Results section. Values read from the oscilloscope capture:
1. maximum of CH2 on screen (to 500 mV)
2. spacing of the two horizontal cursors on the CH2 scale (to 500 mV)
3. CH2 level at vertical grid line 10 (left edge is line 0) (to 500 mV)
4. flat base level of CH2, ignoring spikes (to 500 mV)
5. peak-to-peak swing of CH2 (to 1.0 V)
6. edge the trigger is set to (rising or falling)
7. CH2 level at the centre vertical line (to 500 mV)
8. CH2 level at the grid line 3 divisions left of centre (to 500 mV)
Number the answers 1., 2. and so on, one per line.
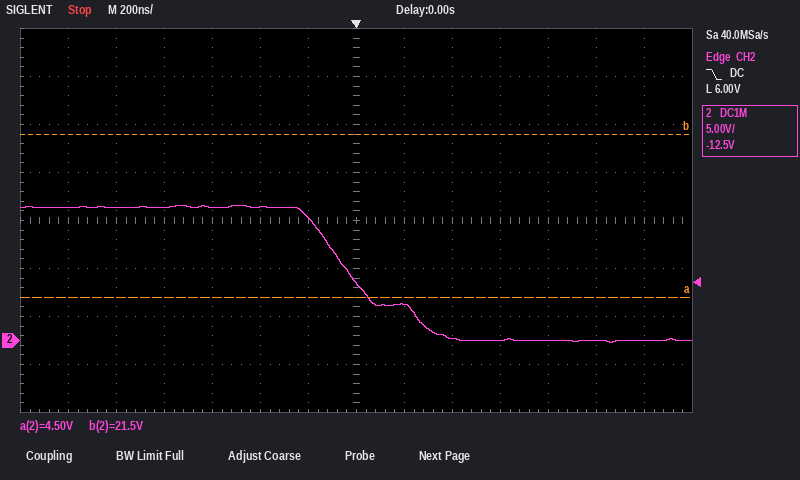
1. 14.0 V
2. 17.0 V
3. 0.0 V
4. 0.0 V
5. 14.0 V
6. falling
7. 6.0 V
8. 14.0 V
